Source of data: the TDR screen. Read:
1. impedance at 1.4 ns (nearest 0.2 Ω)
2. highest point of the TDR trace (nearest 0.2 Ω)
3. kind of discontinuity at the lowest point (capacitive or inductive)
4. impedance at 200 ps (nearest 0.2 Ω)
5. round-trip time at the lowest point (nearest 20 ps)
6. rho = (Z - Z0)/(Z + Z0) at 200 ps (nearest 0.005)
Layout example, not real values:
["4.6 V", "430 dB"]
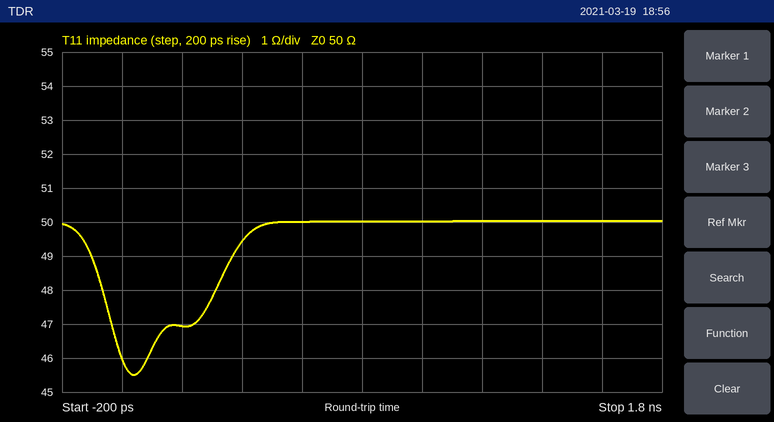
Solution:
["50.0 Ω", "50.0 Ω", "capacitive", "47.0 Ω", "40 ps", "-0.030"]
